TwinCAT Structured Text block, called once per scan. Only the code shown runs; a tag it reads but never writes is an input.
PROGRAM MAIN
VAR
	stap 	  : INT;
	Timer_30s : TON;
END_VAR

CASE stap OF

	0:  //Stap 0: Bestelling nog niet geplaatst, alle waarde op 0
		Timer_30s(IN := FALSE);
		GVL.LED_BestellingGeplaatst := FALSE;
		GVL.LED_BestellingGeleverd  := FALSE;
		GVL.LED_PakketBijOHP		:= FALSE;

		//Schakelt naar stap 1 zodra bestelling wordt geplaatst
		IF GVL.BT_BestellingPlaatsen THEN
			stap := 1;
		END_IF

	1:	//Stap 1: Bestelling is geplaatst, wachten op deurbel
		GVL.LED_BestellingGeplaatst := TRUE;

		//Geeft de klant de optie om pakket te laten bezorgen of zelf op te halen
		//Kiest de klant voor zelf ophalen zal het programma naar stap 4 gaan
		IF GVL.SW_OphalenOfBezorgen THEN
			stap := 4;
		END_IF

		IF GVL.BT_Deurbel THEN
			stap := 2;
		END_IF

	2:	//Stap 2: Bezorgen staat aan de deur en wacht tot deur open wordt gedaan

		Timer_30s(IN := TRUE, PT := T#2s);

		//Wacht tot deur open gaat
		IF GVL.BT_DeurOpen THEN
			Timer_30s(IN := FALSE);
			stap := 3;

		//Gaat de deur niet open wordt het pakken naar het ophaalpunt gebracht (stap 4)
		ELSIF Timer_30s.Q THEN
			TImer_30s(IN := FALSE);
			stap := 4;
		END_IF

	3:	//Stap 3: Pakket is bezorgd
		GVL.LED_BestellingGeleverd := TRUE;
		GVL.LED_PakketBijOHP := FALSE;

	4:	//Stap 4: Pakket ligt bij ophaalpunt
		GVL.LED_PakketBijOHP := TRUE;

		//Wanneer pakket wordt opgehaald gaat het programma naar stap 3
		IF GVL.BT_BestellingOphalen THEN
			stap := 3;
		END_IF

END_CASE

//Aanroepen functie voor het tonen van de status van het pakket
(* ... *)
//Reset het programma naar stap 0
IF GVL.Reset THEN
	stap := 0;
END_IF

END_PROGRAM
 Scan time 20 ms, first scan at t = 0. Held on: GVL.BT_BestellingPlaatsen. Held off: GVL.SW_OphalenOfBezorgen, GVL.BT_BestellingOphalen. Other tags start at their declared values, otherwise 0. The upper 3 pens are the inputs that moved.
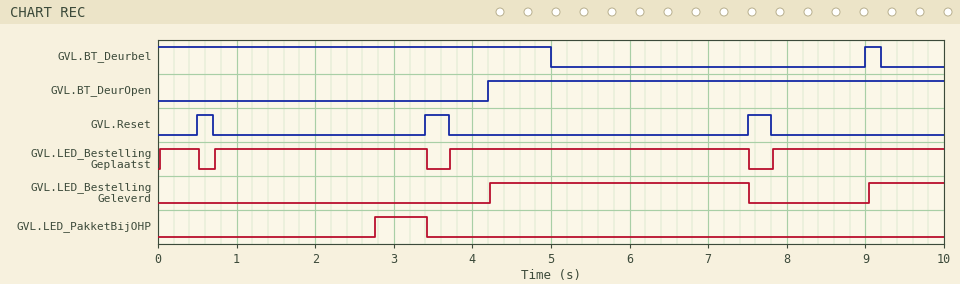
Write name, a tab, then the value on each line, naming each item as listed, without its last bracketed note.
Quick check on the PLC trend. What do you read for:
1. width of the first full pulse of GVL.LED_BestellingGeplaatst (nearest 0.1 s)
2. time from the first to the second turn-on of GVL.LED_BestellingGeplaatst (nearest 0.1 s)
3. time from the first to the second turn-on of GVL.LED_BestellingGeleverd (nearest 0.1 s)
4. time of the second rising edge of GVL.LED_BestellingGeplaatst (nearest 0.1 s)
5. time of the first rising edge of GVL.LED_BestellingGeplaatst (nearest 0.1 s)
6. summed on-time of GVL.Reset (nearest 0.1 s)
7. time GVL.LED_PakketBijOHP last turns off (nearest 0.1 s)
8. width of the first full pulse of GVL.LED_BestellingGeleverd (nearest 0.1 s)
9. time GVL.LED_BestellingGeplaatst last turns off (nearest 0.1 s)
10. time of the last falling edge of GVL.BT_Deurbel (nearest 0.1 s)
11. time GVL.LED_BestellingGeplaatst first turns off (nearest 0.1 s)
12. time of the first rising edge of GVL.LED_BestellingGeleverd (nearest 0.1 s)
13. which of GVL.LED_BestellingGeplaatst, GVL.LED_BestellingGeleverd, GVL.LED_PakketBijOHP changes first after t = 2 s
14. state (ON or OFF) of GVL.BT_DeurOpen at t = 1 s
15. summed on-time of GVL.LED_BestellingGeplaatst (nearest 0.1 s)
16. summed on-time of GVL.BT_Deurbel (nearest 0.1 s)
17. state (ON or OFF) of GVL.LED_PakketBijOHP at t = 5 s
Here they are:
width of the first full pulse of GVL.LED_BestellingGeplaatst	0.5 s
time from the first to the second turn-on of GVL.LED_BestellingGeplaatst	0.7 s
time from the first to the second turn-on of GVL.LED_BestellingGeleverd	4.8 s
time of the second rising edge of GVL.LED_BestellingGeplaatst	0.7 s
time of the first rising edge of GVL.LED_BestellingGeplaatst	0.0 s
summed on-time of GVL.Reset	0.8 s
time GVL.LED_PakketBijOHP last turns off	3.4 s
width of the first full pulse of GVL.LED_BestellingGeleverd	3.3 s
time GVL.LED_BestellingGeplaatst last turns off	7.5 s
time of the last falling edge of GVL.BT_Deurbel	9.2 s
time GVL.LED_BestellingGeplaatst first turns off	0.5 s
time of the first rising edge of GVL.LED_BestellingGeleverd	4.2 s
which of GVL.LED_BestellingGeplaatst, GVL.LED_BestellingGeleverd, GVL.LED_PakketBijOHP changes first after t = 2 s	GVL.LED_PakketBijOHP
state (ON or OFF) of GVL.BT_DeurOpen at t = 1 s	OFF
summed on-time of GVL.LED_BestellingGeplaatst	9.2 s
summed on-time of GVL.BT_Deurbel	5.2 s
state (ON or OFF) of GVL.LED_PakketBijOHP at t = 5 s	OFF
